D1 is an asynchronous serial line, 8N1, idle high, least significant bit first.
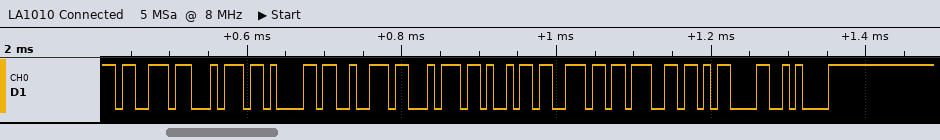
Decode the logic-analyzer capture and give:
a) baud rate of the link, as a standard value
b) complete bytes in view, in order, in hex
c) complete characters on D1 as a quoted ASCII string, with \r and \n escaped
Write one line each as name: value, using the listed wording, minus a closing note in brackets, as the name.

baud rate of the link, as a standard value: 115200 baud
complete bytes in view, in order, in hex: 0x73 0x74 0x61 0x72 0x74 0x69 0x6E 0x67 0x0D 0x0A
complete characters on D1 as a quoted ASCII string, with \r and \n escaped: "starting\r\n"
